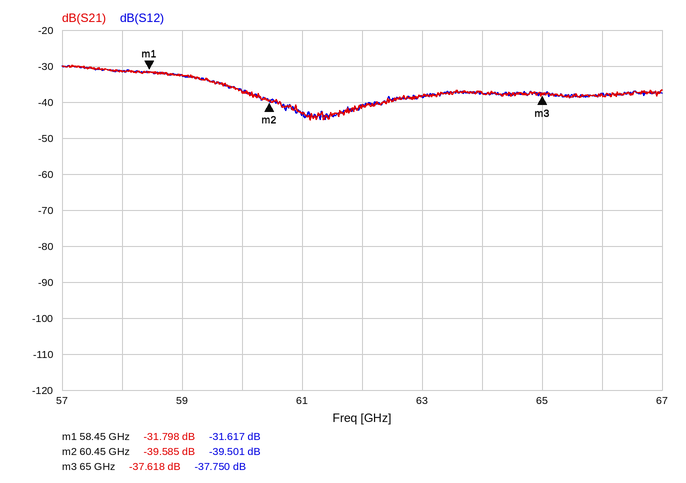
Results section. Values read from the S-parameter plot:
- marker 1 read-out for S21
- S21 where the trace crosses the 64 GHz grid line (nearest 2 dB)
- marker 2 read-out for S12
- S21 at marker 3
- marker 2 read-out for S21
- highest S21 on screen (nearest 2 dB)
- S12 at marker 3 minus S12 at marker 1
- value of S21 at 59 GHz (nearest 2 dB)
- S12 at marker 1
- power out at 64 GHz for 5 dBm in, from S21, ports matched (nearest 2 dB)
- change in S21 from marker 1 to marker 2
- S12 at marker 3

-31.798 dB
-38 dB
-39.501 dB
-37.618 dB
-39.585 dB
-30 dB
-6.133 dB
-32 dB
-31.617 dB
-32 dBm
-7.787 dB
-37.750 dB
